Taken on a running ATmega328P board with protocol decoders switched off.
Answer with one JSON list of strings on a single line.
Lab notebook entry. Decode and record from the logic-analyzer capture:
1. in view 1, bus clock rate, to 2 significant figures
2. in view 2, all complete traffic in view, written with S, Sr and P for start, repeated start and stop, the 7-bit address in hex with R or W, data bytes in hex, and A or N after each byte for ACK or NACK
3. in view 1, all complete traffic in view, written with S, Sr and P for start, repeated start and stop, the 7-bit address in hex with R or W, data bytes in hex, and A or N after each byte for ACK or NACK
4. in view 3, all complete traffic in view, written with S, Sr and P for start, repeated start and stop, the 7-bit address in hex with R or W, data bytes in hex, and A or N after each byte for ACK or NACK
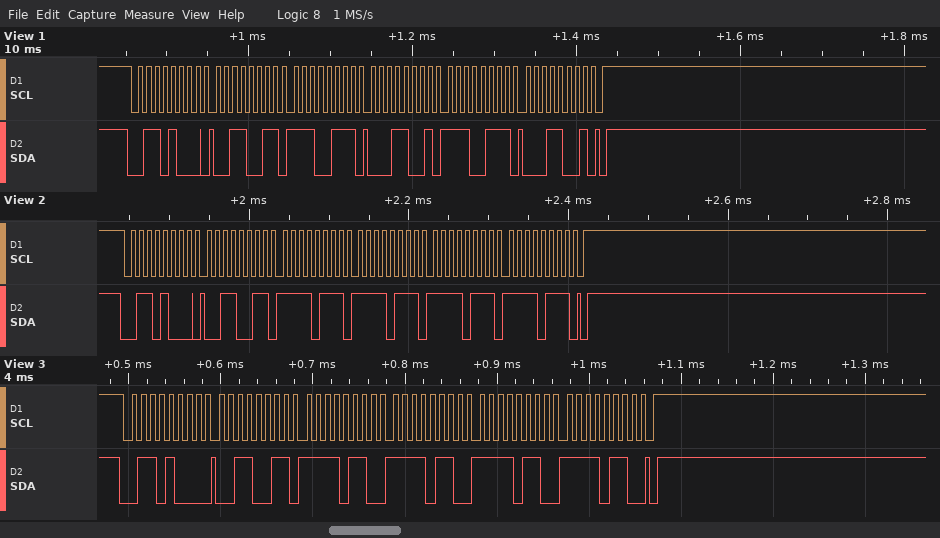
["100 kHz", "S 34W A 33 A F7 A F7 A F7 A F7 A P", "S 34W A 33 A E7 A 19 A E7 A 19 A P", "S 34W A 33 A F6 A F6 A F6 A F6 A P"]
